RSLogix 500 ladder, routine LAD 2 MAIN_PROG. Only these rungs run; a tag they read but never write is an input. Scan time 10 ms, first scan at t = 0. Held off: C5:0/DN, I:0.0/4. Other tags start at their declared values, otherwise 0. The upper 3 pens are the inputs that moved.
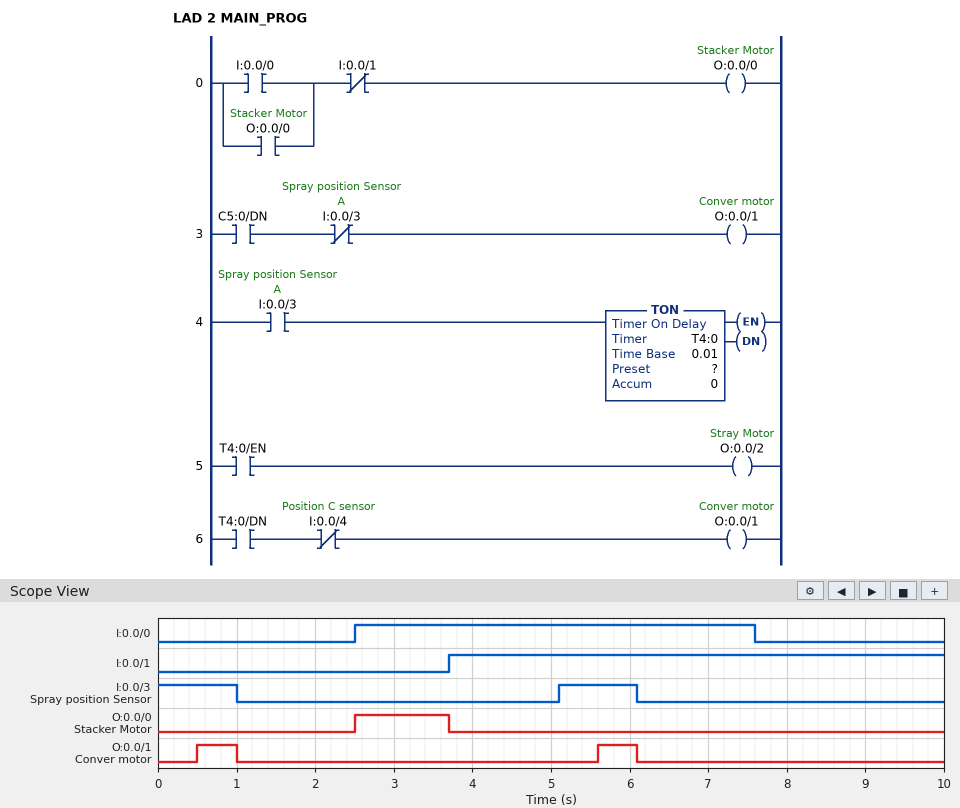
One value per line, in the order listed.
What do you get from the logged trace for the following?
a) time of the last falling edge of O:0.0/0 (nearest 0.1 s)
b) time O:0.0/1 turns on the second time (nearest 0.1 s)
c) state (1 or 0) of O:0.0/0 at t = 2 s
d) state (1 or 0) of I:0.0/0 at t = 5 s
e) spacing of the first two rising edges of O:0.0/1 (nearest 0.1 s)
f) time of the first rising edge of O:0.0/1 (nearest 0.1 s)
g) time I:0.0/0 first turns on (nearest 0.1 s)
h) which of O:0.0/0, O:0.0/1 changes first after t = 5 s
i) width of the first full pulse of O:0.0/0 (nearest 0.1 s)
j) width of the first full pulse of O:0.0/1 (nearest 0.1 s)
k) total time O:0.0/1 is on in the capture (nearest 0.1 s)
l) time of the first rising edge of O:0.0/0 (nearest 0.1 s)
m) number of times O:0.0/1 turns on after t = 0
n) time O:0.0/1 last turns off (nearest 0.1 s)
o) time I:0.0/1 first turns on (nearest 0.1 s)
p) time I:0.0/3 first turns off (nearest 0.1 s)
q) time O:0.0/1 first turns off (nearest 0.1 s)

3.7 s
5.6 s
0
1
5.1 s
0.5 s
2.5 s
O:0.0/1
1.2 s
0.5 s
1.0 s
2.5 s
2
6.1 s
3.7 s
1.0 s
1.0 s
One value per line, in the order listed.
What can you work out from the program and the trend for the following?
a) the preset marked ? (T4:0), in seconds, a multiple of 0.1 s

0.5 s
